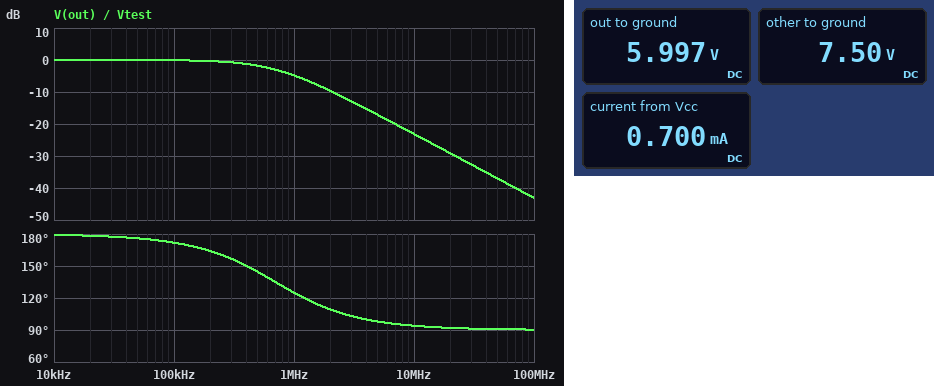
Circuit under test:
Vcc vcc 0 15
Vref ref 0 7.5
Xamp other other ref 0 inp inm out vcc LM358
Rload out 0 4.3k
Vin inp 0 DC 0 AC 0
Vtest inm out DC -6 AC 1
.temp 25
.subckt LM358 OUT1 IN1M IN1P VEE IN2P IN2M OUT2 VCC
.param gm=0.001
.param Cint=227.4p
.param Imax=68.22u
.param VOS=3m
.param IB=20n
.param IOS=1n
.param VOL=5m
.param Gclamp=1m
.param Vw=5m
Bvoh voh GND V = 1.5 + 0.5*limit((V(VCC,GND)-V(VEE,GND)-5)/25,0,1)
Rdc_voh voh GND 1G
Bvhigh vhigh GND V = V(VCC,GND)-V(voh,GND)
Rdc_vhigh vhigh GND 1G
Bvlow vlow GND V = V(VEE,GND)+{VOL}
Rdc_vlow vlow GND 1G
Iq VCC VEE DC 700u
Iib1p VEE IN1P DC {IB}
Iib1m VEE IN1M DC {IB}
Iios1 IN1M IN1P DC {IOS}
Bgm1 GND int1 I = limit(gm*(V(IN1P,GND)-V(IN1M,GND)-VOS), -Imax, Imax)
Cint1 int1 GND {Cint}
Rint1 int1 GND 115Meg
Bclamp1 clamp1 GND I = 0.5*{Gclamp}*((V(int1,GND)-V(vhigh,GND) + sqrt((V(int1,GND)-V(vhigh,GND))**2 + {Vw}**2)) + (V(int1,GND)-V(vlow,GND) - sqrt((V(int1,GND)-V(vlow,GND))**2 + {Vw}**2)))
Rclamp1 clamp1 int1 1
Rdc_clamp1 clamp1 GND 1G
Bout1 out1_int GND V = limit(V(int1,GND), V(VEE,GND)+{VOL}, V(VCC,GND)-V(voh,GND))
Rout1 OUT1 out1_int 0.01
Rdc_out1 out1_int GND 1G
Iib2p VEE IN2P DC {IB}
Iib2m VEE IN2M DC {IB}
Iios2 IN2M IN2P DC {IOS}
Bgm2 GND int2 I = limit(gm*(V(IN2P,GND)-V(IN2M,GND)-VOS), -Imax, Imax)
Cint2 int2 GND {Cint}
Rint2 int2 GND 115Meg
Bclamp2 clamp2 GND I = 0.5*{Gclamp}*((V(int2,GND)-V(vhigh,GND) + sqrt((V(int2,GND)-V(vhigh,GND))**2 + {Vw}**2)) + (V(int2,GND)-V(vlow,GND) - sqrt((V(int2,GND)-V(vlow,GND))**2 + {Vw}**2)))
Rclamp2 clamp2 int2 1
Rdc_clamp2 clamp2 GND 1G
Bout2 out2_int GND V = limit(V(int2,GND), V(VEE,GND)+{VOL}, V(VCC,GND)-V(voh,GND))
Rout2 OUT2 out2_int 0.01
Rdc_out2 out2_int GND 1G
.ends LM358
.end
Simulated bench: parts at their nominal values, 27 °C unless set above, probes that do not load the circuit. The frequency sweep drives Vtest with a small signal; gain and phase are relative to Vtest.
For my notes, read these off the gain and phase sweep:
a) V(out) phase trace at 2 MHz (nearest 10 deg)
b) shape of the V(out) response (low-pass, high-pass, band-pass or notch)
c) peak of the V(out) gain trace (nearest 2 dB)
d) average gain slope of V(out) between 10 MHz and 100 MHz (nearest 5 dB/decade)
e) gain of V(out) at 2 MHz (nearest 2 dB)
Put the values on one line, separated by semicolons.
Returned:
110 deg; low-pass; 0 dB; -20 dB/decade; -10 dB
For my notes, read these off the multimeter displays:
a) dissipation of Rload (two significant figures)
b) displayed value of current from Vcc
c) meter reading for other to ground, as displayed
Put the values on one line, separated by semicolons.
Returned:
8.4 mW; 0.700 mA; 7.50 V
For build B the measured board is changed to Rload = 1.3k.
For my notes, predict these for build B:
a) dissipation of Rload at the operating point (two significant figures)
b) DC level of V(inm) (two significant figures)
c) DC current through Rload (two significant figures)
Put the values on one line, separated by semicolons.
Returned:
28 mW; -3.1 mV; 4.6 mA
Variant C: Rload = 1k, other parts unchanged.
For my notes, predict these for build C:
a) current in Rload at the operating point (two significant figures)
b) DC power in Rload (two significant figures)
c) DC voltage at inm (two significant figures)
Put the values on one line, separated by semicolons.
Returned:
6.0 mA; 36 mW; -3.1 mV
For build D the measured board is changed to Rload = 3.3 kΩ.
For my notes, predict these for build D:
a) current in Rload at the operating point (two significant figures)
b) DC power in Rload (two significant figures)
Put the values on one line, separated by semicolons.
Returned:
1.8 mA; 11 mW
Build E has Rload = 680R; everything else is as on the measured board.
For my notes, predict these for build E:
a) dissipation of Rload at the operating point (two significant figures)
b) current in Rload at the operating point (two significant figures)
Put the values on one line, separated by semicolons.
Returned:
53 mW; 8.8 mA
